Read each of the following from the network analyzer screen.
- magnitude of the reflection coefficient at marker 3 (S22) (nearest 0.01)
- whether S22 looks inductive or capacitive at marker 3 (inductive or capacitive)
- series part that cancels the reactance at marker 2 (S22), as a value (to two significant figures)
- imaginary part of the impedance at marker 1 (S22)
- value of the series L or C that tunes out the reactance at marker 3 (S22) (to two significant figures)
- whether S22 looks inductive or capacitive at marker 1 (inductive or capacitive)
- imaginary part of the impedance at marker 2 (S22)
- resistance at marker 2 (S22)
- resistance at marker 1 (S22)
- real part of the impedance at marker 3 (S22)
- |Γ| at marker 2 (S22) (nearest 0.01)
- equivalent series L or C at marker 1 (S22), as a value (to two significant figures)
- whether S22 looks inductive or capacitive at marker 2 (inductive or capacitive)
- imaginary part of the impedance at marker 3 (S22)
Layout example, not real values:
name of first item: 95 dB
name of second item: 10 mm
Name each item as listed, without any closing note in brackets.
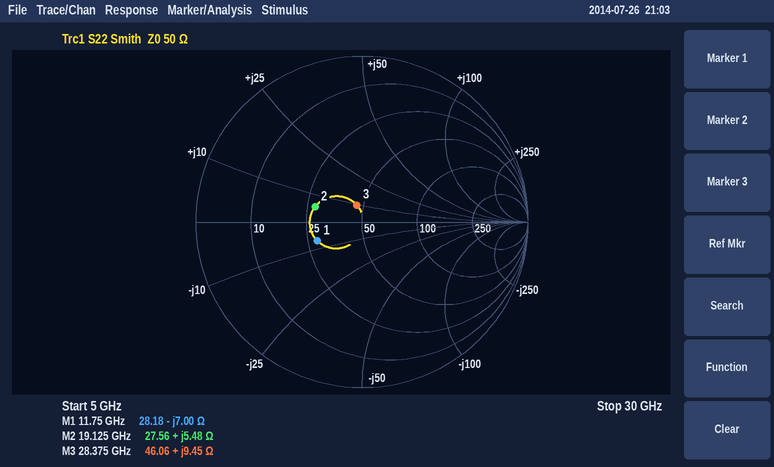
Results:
magnitude of the reflection coefficient at marker 3 (S22): 0.11
whether S22 looks inductive or capacitive at marker 3: inductive
series part that cancels the reactance at marker 2 (S22), as a value: 1.5 pF
imaginary part of the impedance at marker 1: -7.00 Ω
value of the series L or C that tunes out the reactance at marker 3 (S22): 590 fF
whether S22 looks inductive or capacitive at marker 1: capacitive
imaginary part of the impedance at marker 2: +5.48 Ω
resistance at marker 2: 27.56 Ω
resistance at marker 1: 28.18 Ω
real part of the impedance at marker 3: 46.06 Ω
|Γ| at marker 2 (S22): 0.30
equivalent series L or C at marker 1 (S22), as a value: 1.9 pF
whether S22 looks inductive or capacitive at marker 2: inductive
imaginary part of the impedance at marker 3: +9.45 Ω
